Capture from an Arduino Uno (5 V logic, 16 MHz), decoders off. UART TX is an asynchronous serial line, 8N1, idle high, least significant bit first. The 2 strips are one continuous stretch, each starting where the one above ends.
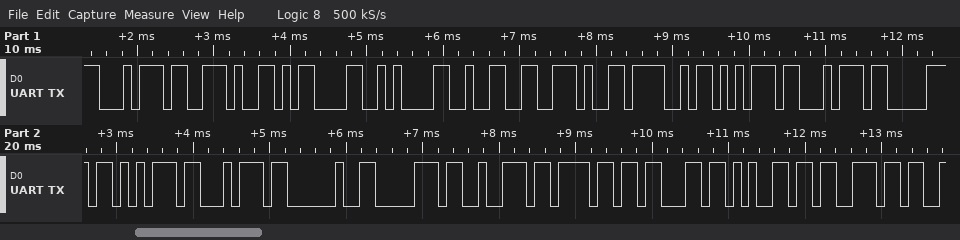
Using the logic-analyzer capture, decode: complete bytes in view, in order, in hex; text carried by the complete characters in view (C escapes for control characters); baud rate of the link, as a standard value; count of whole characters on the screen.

0x74 0x2E 0x0D 0x0A 0x32 0x2E 0x4F 0x75 0x74 0x70 0x75 0x74 0x20 0x70 0x72 0x6F 0x63 0x65 0x73
"t.\r\n2.Output proces"
9600 baud
19
